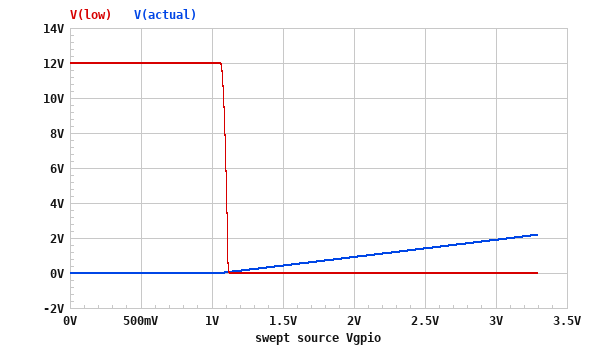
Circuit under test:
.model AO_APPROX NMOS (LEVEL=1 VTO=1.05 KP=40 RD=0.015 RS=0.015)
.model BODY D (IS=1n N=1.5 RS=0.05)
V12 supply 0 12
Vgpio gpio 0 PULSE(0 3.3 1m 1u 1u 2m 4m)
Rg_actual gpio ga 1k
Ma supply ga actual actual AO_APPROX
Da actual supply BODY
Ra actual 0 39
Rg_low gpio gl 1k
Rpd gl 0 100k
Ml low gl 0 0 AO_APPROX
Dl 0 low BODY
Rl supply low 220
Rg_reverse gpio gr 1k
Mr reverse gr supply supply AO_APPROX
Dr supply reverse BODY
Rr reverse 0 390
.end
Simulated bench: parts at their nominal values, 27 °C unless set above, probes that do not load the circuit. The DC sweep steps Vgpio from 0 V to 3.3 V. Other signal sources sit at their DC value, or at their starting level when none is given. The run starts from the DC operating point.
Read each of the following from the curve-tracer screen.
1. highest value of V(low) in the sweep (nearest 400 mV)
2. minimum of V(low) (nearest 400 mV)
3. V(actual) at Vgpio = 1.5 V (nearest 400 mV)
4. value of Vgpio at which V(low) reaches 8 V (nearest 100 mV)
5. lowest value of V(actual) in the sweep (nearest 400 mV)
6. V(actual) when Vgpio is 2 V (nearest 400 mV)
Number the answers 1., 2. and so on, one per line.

1. 12.0 V
2. 0 V
3. 400 mV
4. 1.1 V
5. 0 V
6. 800 mV
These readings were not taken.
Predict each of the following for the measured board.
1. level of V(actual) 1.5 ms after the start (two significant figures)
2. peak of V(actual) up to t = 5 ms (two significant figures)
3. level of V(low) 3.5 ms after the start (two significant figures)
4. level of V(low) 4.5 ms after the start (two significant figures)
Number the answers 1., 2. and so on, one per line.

1. 2.2 V
2. 2.2 V
3. 12 V
4. 12 V
